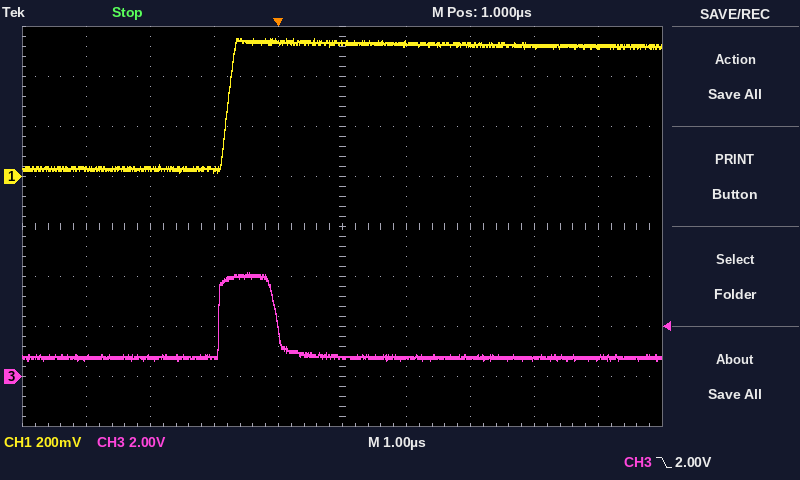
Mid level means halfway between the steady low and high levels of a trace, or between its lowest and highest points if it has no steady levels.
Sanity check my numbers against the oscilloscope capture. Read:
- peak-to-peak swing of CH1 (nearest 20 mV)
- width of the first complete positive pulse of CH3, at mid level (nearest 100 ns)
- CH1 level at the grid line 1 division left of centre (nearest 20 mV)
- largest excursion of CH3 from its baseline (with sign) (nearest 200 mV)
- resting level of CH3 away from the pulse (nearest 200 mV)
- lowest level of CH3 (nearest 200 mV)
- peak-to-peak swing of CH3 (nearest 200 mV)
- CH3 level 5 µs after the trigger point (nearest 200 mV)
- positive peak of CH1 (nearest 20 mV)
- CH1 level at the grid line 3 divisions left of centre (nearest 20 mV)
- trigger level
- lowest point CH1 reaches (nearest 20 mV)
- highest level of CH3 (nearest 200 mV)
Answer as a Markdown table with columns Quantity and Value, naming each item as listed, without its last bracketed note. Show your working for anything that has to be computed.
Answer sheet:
| Quantity | Value |
|---|---|
| peak-to-peak swing of CH1 | 560 mV − (20 mV) = 540 mV |
| width of the first complete positive pulse of CH3, at mid level | 900 ns |
| CH1 level at the grid line 1 division left of centre | 540 mV |
| largest excursion of CH3 from its baseline (with sign) | 4.2 V − (800 mV) = +3.4 V |
| resting level of CH3 away from the pulse | 800 mV |
| lowest level of CH3 | 600 mV |
| peak-to-peak swing of CH3 | 4.2 V − (600 mV) = 3.6 V |
| CH3 level 5 µs after the trigger point | 800 mV |
| positive peak of CH1 | 560 mV |
| CH1 level at the grid line 3 divisions left of centre | 40 mV |
| trigger level | 2.00 V |
| lowest point CH1 reaches | 20 mV |
| highest level of CH3 | 4.2 V |
